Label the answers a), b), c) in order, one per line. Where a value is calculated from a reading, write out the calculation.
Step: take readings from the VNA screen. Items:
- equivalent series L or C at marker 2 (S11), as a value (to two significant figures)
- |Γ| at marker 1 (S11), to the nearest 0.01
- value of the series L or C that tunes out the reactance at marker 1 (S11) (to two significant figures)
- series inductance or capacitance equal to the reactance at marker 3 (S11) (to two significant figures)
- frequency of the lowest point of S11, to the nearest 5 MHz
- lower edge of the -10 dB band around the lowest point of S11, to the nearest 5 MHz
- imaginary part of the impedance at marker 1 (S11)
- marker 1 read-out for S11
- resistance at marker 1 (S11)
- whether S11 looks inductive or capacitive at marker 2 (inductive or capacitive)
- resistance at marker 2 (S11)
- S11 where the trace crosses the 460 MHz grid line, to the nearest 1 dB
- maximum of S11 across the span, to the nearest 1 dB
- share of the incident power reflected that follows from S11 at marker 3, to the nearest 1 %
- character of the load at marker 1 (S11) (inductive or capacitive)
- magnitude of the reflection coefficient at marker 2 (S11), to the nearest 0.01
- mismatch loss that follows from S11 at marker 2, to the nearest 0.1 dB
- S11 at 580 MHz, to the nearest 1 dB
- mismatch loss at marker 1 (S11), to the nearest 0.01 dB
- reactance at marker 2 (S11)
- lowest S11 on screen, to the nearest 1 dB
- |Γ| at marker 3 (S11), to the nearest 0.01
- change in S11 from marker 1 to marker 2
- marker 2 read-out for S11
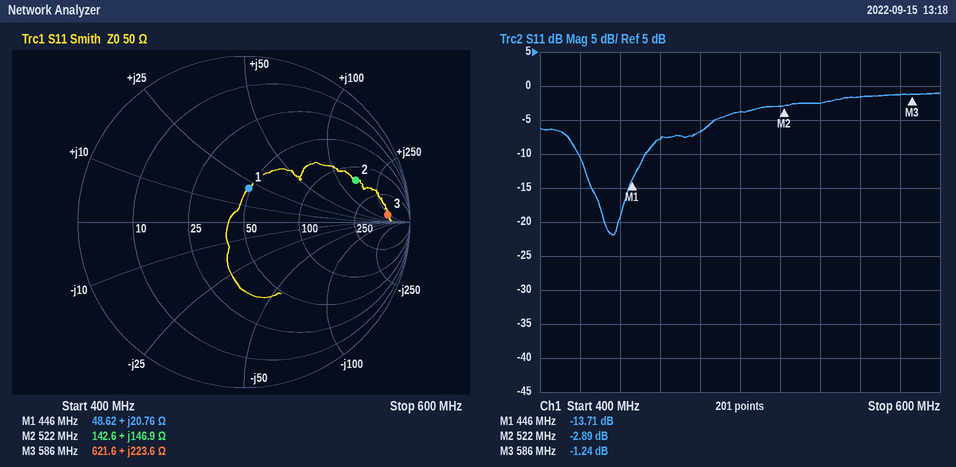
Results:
a) L = 146.9 Ω/(2π × 522 MHz) ≈ 45 nH
b) 0.21
c) C = 1/(2π × 446 MHz × 20.76 Ω) ≈ 17 pF
d) L = 223.6 Ω/(2π × 586 MHz) ≈ 61 nH
e) 435 MHz
f) 420 MHz
g) +20.76 Ω
h) -13.71 dB
i) 48.62 Ω
j) inductive
k) 142.6 Ω
l) -8 dB
m) -1 dB
n) 10^(-1.24/10) ≈ 75 %
o) inductive
p) 0.72
q) −10 log10(1 − 10^(-2.89/10)) ≈ 3.1 dB
r) -1 dB
s) −10 log10(1 − 10^(-13.71/10)) ≈ 0.19 dB
t) +146.9 Ω
u) -22 dB
v) 0.87
w) -2.89 − (-13.71) = 10.82 dB
x) -2.89 dB
